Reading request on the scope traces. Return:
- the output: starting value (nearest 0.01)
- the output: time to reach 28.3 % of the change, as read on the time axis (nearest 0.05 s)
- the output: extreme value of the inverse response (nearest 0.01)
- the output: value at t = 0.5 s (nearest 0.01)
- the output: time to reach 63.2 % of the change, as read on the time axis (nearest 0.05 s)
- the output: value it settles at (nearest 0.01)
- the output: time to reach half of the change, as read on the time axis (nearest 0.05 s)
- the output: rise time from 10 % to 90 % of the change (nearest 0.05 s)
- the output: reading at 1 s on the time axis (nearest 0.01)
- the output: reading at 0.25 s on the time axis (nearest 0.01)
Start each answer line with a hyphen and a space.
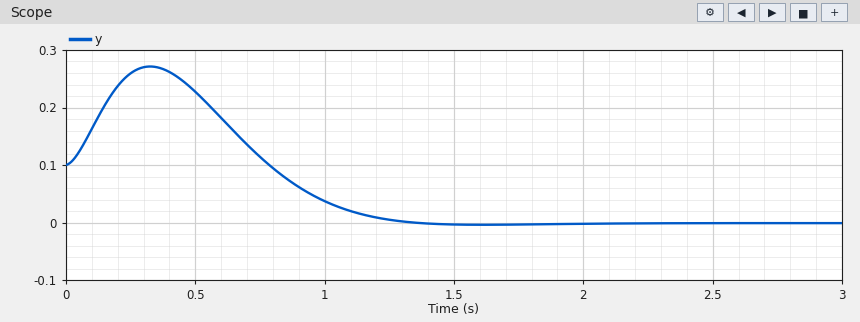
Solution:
- 0.10
- 0.85 s
- 0.27
- 0.23
- 1.00 s
- 0.00
- 0.95 s
- 0.40 s
- 0.04
- 0.26
